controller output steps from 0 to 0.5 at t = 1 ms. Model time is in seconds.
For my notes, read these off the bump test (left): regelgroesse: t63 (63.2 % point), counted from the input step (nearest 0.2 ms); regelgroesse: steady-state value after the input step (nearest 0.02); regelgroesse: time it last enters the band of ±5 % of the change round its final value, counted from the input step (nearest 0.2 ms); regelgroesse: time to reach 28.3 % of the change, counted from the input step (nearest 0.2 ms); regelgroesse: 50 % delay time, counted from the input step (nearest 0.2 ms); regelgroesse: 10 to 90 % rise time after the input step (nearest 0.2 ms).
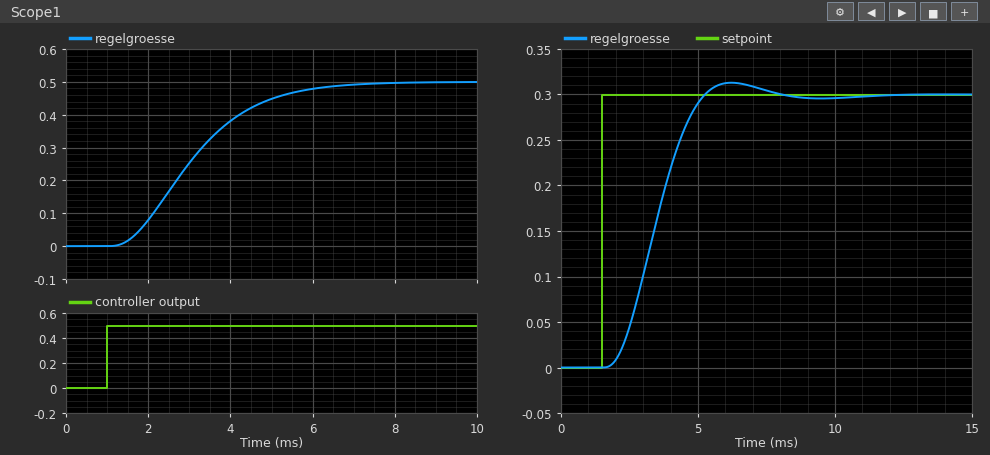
2.4 ms
0.50
4.8 ms
1.4 ms
2.0 ms
3.2 ms
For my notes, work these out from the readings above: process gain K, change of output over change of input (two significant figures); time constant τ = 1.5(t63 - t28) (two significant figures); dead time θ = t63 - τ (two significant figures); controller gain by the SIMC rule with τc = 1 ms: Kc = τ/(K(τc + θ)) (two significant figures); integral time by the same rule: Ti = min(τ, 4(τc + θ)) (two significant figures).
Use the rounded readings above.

1.0
1.5 ms
0.90 ms
0.79
1.5 ms
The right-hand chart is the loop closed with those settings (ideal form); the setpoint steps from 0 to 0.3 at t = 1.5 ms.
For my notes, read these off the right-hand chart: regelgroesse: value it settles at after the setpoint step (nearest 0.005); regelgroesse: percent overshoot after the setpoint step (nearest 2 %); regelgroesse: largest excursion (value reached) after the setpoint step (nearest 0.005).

0.300
4 %
0.315
